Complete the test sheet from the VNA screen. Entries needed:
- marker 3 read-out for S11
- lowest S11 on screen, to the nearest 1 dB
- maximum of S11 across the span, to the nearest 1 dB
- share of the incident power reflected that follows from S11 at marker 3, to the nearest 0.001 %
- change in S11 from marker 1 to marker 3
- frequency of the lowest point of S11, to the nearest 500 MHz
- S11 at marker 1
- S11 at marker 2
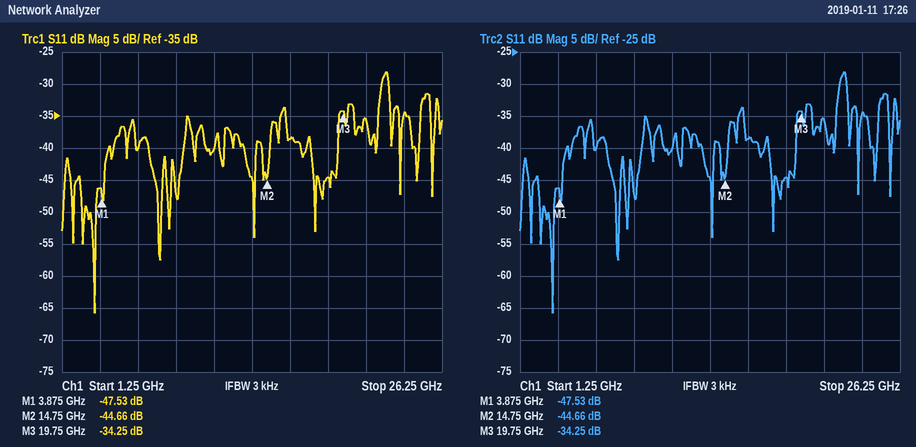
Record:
-34.25 dB
-66 dB
-28 dB
0.038 %
13.28 dB
3.5 GHz
-47.53 dB
-44.66 dB
